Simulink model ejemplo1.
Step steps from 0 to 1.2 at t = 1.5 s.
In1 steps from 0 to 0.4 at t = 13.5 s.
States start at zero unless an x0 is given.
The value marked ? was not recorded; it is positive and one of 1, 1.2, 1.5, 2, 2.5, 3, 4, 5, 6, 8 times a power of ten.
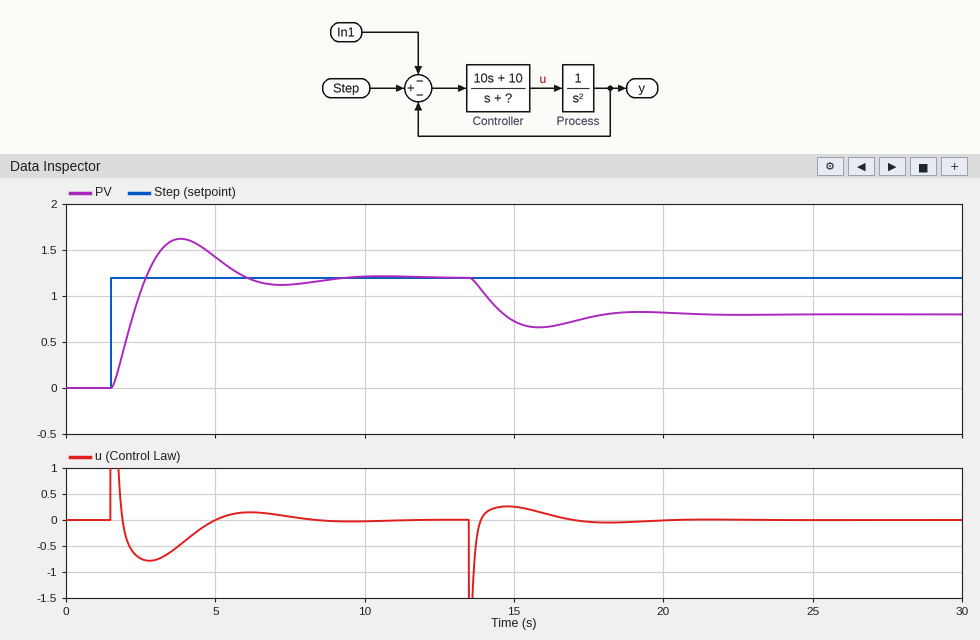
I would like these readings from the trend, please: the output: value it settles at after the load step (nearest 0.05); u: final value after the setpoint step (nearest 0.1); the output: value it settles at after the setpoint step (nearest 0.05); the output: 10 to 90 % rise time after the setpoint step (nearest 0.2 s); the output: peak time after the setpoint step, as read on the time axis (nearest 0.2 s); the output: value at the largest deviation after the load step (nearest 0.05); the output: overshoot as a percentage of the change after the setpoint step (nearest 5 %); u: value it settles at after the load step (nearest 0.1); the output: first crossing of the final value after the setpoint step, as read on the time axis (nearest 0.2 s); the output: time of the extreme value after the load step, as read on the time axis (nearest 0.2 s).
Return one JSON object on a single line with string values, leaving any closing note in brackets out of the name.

{"the output: value it settles at after the load step": "0.80", "u: final value after the setpoint step": "0.0", "the output: value it settles at after the setpoint step": "1.20", "the output: 10 to 90 % rise time after the setpoint step": "0.8 s", "the output: peak time after the setpoint step, as read on the time axis": "3.8 s", "the output: value at the largest deviation after the load step": "0.65", "the output: overshoot as a percentage of the change after the setpoint step": "35 %", "u: value it settles at after the load step": "0.0", "the output: first crossing of the final value after the setpoint step, as read on the time axis": "2.6 s", "the output: time of the extreme value after the load step, as read on the time axis": "15.8 s"}
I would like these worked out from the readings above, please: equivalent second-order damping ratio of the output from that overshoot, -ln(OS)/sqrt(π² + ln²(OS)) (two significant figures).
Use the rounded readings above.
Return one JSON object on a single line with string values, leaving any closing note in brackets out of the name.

{"equivalent second-order damping ratio of the output from that overshoot, -ln(OS)/sqrt(π² + ln²(OS))": "0.32"}
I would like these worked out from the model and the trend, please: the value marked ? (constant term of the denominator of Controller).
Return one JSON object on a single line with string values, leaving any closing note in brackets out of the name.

{"the value marked ?": "10"}
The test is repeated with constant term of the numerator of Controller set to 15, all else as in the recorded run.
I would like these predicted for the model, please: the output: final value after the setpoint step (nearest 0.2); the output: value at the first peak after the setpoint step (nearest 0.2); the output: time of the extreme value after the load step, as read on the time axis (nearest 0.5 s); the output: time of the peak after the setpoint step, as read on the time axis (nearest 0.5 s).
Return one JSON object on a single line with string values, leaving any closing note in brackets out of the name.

{"the output: final value after the setpoint step": "1.2", "the output: value at the first peak after the setpoint step": "1.8", "the output: time of the extreme value after the load step, as read on the time axis": "15.5 s", "the output: time of the peak after the setpoint step, as read on the time axis": "3.5 s"}
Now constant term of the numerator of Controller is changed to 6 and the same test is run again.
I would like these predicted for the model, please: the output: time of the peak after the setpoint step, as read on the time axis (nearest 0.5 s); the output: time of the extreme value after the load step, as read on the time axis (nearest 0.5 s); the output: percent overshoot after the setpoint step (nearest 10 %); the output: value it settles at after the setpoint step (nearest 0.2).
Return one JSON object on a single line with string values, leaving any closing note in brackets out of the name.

{"the output: time of the peak after the setpoint step, as read on the time axis": "4.5 s", "the output: time of the extreme value after the load step, as read on the time axis": "16.5 s", "the output: percent overshoot after the setpoint step": "30 %", "the output: value it settles at after the setpoint step": "1.2"}
